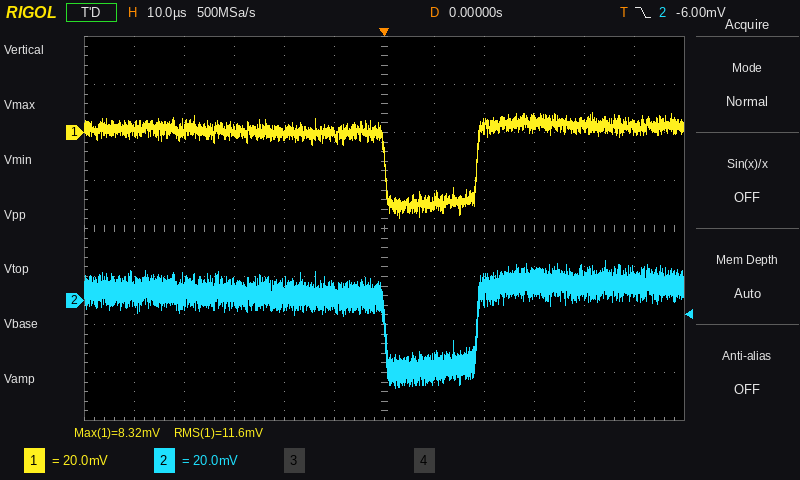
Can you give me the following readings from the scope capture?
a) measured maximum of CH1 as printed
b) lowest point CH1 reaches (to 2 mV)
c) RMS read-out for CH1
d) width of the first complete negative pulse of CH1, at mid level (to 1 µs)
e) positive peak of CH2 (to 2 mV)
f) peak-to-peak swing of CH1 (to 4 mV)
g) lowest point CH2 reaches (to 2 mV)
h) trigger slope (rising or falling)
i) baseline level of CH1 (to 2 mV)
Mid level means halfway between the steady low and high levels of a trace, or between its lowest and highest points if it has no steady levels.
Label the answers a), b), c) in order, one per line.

a) 8.32 mV
b) -36 mV
c) 11.6 mV
d) 18 µs
e) 16 mV
f) 44 mV
g) -36 mV
h) falling
i) 2 mV
